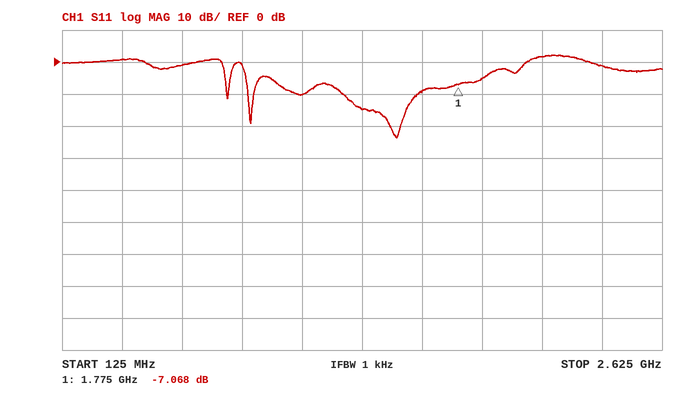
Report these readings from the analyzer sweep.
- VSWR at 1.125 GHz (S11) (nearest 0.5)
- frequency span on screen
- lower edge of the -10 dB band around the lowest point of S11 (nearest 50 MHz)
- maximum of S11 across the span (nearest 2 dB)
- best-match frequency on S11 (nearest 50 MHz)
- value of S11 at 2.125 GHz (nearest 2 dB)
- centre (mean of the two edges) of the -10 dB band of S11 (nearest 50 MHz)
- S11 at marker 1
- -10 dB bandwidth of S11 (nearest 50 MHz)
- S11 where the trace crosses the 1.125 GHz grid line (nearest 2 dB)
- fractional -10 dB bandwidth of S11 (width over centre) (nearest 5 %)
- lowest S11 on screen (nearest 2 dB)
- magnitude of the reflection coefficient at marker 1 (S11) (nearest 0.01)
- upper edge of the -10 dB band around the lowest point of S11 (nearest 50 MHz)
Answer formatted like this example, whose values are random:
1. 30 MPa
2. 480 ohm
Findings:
1. 2.0
2. 2.5 GHz
3. 1.30 GHz
4. 2 dB
5. 1.50 GHz
6. 2 dB
7. 1.45 GHz
8. -7.068 dB
9. 300 MHz
10. -10 dB
11. 20 %
12. -24 dB
13. 0.44
14. 1.60 GHz
